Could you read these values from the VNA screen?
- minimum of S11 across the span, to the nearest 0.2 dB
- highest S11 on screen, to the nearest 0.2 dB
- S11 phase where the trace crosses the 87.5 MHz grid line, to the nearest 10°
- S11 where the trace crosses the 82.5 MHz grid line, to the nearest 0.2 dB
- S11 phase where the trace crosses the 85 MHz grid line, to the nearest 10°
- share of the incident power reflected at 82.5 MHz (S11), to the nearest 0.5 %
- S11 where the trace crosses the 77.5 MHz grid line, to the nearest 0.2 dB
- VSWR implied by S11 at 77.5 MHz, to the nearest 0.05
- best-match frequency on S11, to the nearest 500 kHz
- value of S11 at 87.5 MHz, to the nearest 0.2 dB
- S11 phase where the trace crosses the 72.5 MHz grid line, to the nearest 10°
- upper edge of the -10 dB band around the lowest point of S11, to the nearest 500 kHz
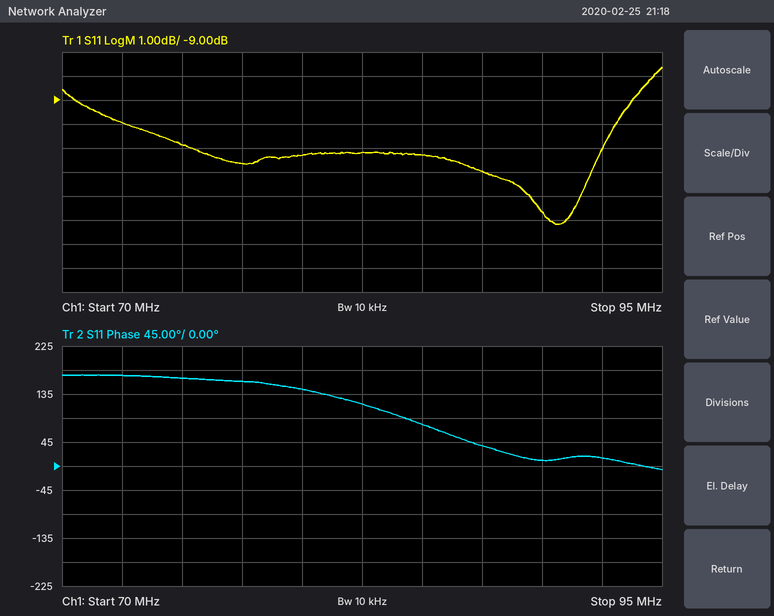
-14.2 dB
-7.6 dB
40°
-11.2 dB
80°
7.5 %
-11.6 dB
1.70
90.5 MHz
-12.0 dB
170°
93.0 MHz
